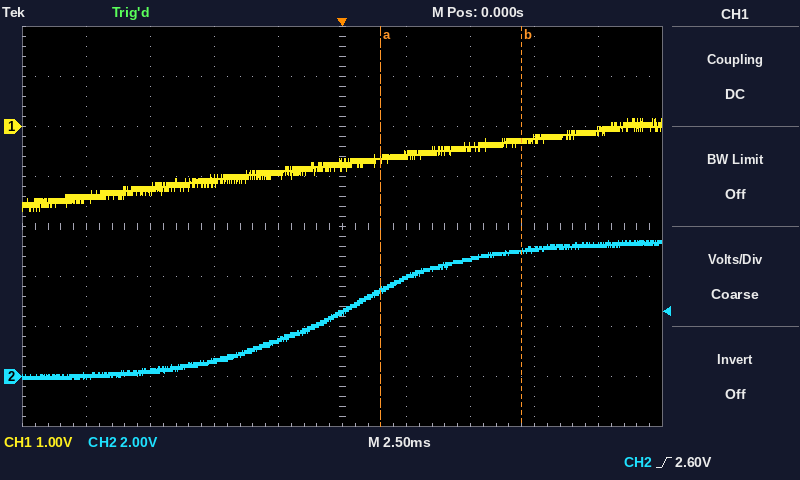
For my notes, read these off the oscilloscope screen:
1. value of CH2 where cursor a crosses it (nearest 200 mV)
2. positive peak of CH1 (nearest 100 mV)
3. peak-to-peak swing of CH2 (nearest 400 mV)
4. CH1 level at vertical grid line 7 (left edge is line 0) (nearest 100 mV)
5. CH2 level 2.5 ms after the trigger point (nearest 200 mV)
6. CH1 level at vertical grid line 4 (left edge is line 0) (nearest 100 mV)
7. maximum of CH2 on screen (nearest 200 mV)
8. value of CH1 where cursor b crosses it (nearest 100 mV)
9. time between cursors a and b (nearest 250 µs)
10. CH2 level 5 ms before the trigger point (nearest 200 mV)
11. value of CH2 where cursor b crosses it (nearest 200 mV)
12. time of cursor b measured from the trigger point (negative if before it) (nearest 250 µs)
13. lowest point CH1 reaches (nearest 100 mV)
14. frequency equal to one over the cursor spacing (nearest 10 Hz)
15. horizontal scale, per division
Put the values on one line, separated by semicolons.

3.4 V; 200 mV; 5.6 V; -400 mV; 4.0 V; -900 mV; 5.4 V; -300 mV; 5.50 ms; 600 mV; 5.0 V; +7.00 ms; -1.7 V; 180 Hz; 2.5 ms
